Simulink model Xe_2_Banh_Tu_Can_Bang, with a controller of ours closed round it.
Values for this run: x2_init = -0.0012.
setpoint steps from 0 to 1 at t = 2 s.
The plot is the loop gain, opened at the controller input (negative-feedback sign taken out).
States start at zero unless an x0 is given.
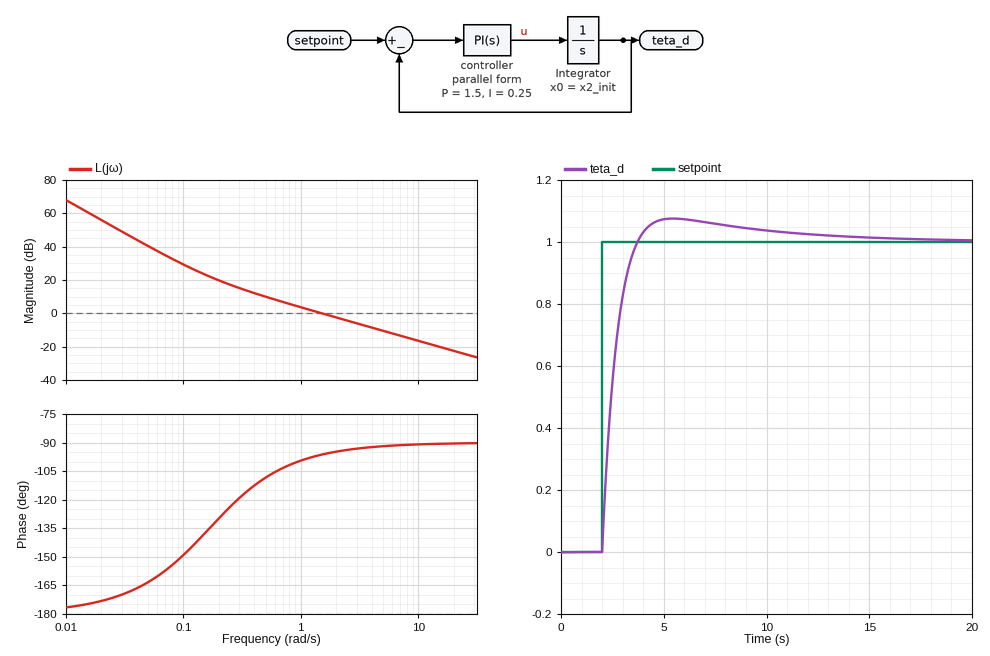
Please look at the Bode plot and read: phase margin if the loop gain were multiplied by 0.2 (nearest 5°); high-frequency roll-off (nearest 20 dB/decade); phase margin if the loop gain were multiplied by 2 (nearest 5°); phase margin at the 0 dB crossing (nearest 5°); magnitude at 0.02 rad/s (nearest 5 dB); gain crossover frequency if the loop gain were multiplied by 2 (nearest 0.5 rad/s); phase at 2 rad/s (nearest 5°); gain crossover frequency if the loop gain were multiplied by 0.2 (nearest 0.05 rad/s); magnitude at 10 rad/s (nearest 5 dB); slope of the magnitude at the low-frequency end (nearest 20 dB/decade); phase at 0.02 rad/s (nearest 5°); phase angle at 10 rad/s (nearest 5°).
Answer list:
65°
-20 dB/decade
85°
85°
55 dB
3.0 rad/s
-95°
0.35 rad/s
-15 dB
-40 dB/decade
-175°
-90°
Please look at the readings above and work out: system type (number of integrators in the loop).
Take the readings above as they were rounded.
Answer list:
2
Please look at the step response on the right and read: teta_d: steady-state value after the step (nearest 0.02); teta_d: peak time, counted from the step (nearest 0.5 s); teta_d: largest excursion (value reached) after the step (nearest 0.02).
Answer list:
1.00
3.5 s
1.08
